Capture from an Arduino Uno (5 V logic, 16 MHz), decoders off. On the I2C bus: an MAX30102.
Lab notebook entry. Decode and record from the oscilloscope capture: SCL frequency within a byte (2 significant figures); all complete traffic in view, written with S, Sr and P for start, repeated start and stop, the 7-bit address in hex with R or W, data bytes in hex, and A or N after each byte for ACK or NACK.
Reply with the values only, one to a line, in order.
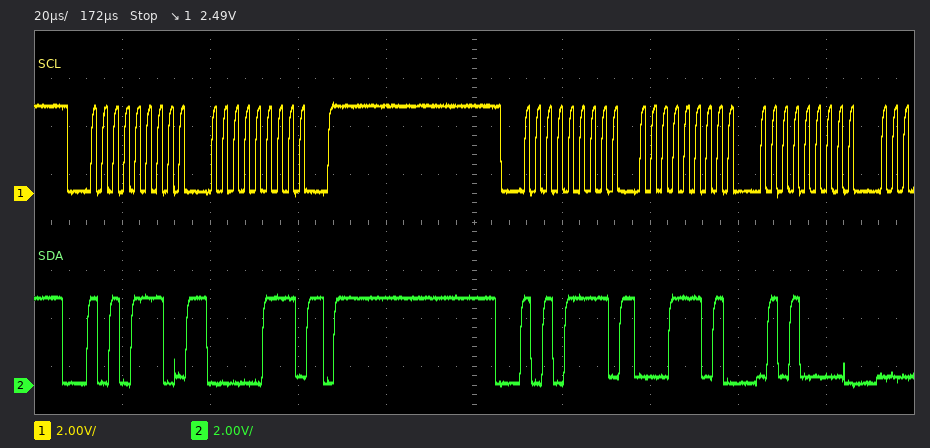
400 kHz
S 57W A 07 A P S 57R A 1D A 50 A
